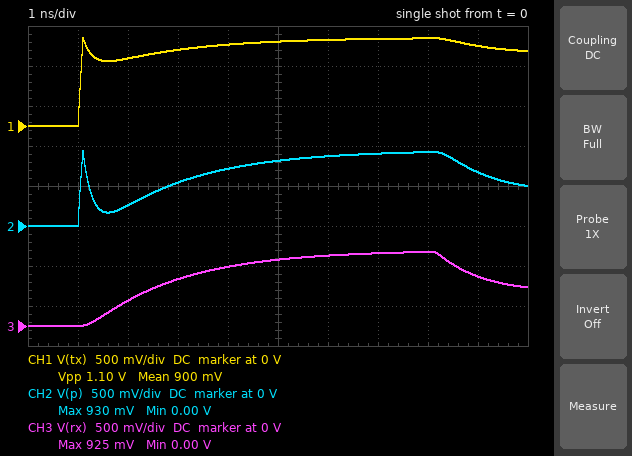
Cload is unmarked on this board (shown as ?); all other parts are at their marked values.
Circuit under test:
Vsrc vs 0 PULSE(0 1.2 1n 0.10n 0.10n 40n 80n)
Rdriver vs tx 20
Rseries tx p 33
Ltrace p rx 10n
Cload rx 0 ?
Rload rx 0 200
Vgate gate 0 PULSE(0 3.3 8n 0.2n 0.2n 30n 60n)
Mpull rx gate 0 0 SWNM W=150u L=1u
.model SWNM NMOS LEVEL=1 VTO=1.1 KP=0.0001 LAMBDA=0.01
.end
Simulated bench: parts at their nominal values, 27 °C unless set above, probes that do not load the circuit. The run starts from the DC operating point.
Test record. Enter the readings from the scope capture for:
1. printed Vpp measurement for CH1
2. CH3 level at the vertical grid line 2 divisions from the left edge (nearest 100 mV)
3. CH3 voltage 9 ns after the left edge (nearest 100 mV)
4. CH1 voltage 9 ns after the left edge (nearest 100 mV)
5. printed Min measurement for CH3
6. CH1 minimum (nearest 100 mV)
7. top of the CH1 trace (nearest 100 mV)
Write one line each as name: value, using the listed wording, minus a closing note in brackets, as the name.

printed Vpp measurement for CH1: 1.10 V
CH3 level at the vertical grid line 2 divisions from the left edge: 300 mV
CH3 voltage 9 ns after the left edge: 600 mV
CH1 voltage 9 ns after the left edge: 1.0 V
printed Min measurement for CH3: 0.00 V
CH1 minimum: 0 V
top of the CH1 trace: 1.1 V
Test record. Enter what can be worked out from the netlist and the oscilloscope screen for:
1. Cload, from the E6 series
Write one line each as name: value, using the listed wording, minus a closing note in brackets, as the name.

Cload, from the E6 series: 47 pF
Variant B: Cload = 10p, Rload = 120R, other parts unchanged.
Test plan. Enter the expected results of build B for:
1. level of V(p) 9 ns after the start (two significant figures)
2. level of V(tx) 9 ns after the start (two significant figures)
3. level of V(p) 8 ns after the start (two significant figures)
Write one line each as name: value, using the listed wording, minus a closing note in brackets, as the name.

level of V(p) 9 ns after the start: 390 mV
level of V(tx) 9 ns after the start: 900 mV
level of V(p) 8 ns after the start: 830 mV
